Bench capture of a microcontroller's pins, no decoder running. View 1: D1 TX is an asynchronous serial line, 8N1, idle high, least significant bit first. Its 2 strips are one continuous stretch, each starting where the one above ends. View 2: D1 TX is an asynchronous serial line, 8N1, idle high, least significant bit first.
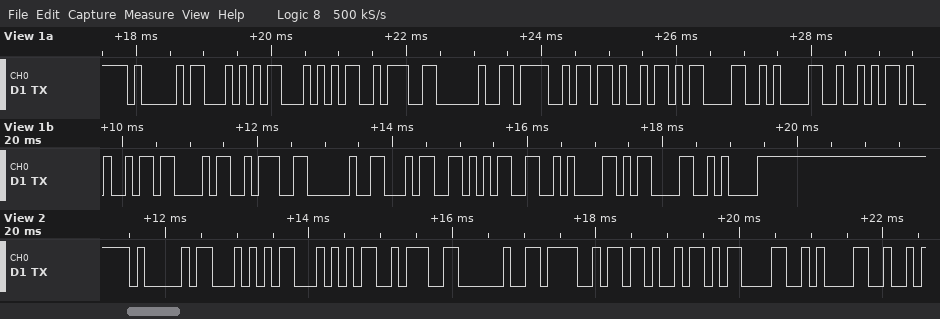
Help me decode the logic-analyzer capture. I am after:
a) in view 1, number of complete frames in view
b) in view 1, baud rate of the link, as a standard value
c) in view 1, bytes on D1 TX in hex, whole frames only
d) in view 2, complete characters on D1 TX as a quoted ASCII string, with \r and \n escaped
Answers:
19
9600 baud
41 54 54 3A 20 4F 4B 0D 0A 52 49 43 3A 20 34 35 0A 0D 0A
"ATT: OK\r\n"
